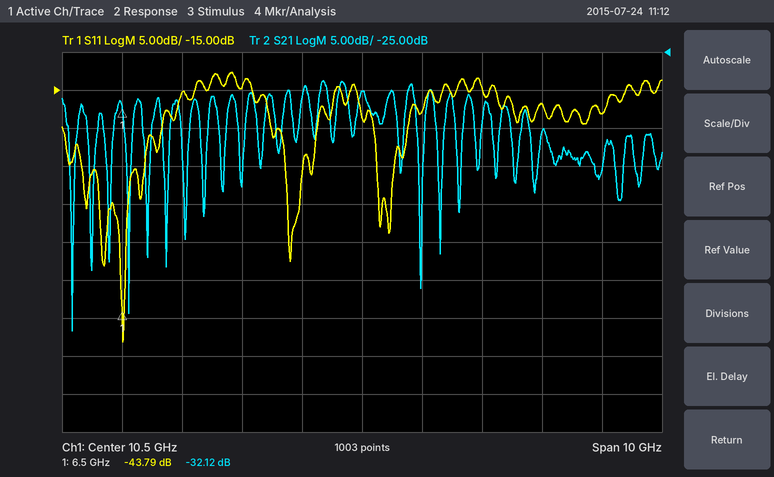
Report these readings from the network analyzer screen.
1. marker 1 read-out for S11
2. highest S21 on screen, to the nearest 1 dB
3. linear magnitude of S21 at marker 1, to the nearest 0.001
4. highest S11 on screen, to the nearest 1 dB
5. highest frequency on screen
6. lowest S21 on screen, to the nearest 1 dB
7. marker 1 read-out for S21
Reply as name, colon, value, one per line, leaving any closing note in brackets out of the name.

marker 1 read-out for S11: -43.79 dB
highest S21 on screen, to the nearest 1 dB: -29 dB
linear magnitude of S21 at marker 1, to the nearest 0.001: 0.025
highest S11 on screen, to the nearest 1 dB: -13 dB
highest frequency on screen: 15.5 GHz
lowest S21 on screen, to the nearest 1 dB: -62 dB
marker 1 read-out for S21: -32.12 dB
